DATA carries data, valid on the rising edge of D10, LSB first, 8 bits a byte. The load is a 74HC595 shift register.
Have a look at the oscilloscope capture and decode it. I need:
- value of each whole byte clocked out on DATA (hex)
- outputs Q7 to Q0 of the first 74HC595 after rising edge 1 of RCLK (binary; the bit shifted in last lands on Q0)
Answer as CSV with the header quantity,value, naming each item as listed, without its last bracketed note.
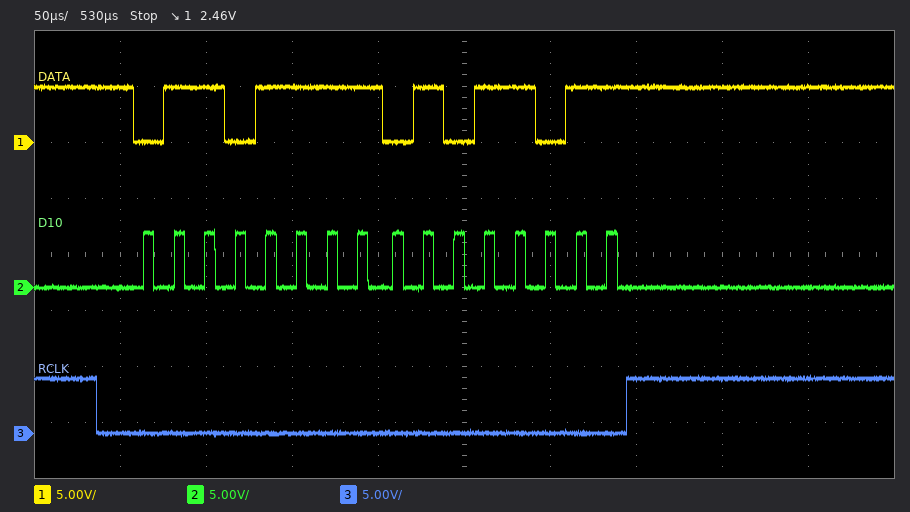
quantity,value
value of each whole byte clocked out on DATA,F6 DA
outputs Q7 to Q0 of the first 74HC595 after rising edge 1 of RCLK,01011011
